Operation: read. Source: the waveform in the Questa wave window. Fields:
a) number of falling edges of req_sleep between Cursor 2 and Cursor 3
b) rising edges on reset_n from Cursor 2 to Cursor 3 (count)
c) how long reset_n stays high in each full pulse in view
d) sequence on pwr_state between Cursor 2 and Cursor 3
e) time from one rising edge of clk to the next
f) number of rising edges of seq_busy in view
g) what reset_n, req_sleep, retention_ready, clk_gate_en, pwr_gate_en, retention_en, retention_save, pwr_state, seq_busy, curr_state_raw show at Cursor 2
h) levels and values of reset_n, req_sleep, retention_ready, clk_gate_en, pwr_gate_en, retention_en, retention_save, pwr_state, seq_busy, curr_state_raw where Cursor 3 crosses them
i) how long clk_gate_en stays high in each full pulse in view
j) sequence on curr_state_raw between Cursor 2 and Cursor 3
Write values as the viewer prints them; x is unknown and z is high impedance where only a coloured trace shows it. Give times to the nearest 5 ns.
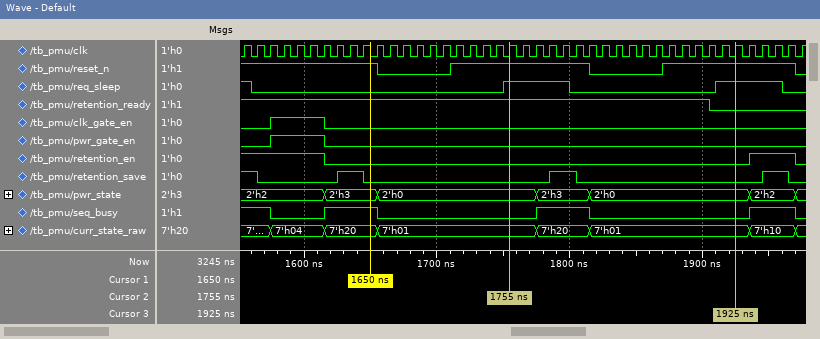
1
1
105 ns, 100 ns
2'h0, 2'h3, 2'h0
10 ns
3
reset_n=1, req_sleep=1, retention_ready=1, clk_gate_en=0, pwr_gate_en=0, retention_en=0, retention_save=0, pwr_state=2'h0, seq_busy=0, curr_state_raw=7'h01
reset_n=1, req_sleep=1, retention_ready=0, clk_gate_en=0, pwr_gate_en=0, retention_en=0, retention_save=0, pwr_state=2'h0, seq_busy=0, curr_state_raw=7'h01
40 ns
7'h01, 7'h20, 7'h01
